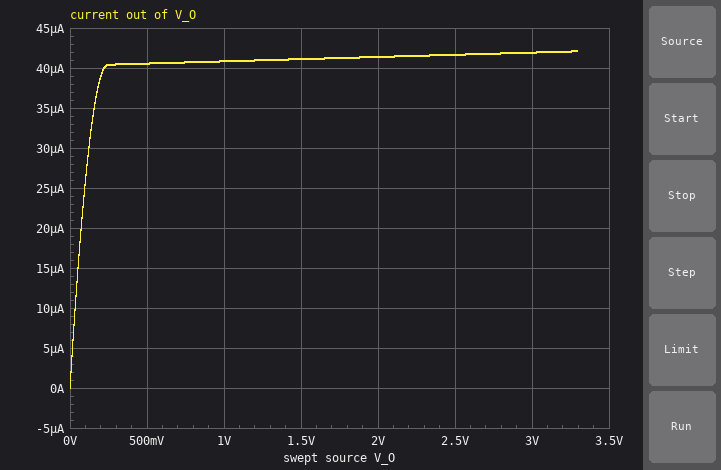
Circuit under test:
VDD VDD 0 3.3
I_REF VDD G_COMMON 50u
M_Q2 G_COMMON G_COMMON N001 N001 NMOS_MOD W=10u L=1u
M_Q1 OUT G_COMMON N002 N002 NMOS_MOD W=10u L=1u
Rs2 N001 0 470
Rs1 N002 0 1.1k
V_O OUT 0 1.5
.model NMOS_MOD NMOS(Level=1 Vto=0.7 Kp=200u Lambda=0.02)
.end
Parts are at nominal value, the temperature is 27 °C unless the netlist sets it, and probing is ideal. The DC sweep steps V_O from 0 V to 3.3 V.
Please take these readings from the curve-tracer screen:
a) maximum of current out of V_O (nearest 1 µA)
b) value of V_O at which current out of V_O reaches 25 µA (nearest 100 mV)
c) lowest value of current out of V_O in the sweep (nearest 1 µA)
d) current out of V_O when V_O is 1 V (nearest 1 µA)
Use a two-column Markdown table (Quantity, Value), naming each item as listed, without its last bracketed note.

| Quantity | Value |
|---|---|
| maximum of current out of V_O | 42 µA |
| value of V_O at which current out of V_O reaches 25 µA | 100 mV |
| lowest value of current out of V_O in the sweep | 0 A |
| current out of V_O when V_O is 1 V | 41 µA |
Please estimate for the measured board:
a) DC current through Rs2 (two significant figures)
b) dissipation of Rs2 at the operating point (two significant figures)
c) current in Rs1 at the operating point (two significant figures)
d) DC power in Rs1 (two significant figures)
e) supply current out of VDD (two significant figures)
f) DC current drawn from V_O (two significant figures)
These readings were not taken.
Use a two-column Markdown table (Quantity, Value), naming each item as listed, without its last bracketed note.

| Quantity | Value |
|---|---|
| DC current through Rs2 | 50 µA |
| dissipation of Rs2 at the operating point | 1.2 µW |
| current in Rs1 at the operating point | 41 µA |
| DC power in Rs1 | 1.9 µW |
| supply current out of VDD | 50 µA |
| DC current drawn from V_O | 41 µA |
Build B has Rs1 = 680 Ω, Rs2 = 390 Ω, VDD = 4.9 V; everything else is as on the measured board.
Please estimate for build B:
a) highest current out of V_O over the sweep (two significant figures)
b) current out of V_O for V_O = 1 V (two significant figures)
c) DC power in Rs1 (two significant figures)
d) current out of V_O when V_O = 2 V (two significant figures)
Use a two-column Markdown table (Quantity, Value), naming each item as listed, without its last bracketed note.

| Quantity | Value |
|---|---|
| highest current out of V_O over the sweep | 47 µA |
| current out of V_O for V_O = 1 V | 45 µA |
| DC power in Rs1 | 1.4 µW |
| current out of V_O when V_O = 2 V | 46 µA |
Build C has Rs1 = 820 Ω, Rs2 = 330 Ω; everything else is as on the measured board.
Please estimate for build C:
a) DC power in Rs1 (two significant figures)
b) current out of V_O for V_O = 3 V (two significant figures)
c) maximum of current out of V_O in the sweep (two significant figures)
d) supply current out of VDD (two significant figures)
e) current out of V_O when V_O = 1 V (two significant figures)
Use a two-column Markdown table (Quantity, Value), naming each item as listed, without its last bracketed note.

| Quantity | Value |
|---|---|
| DC power in Rs1 | 1.5 µW |
| current out of V_O for V_O = 3 V | 43 µA |
| maximum of current out of V_O in the sweep | 44 µA |
| supply current out of VDD | 50 µA |
| current out of V_O when V_O = 1 V | 42 µA |
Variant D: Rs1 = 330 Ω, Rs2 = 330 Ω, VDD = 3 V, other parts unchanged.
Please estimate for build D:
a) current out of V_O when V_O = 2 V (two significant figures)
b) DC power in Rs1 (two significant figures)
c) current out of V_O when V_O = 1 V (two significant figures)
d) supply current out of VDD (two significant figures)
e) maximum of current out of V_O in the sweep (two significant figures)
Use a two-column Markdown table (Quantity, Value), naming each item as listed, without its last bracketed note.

| Quantity | Value |
|---|---|
| current out of V_O when V_O = 2 V | 51 µA |
| DC power in Rs1 | 840 nW |
| current out of V_O when V_O = 1 V | 50 µA |
| supply current out of VDD | 50 µA |
| maximum of current out of V_O in the sweep | 52 µA |
